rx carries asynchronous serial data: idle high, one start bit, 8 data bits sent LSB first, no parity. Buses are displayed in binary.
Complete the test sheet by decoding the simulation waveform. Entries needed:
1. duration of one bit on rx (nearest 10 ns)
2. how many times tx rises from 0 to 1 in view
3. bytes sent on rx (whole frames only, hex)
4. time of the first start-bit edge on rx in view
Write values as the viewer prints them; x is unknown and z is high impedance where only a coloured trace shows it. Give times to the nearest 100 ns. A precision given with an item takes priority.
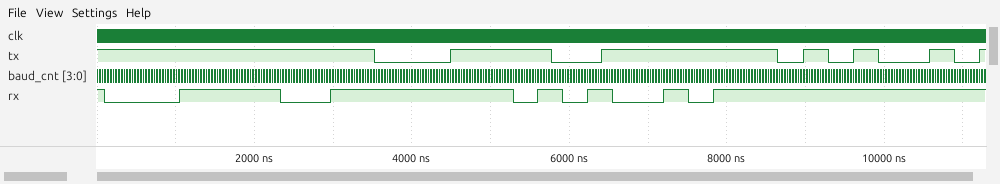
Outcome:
310 ns
6
3C, A5
100 ns
